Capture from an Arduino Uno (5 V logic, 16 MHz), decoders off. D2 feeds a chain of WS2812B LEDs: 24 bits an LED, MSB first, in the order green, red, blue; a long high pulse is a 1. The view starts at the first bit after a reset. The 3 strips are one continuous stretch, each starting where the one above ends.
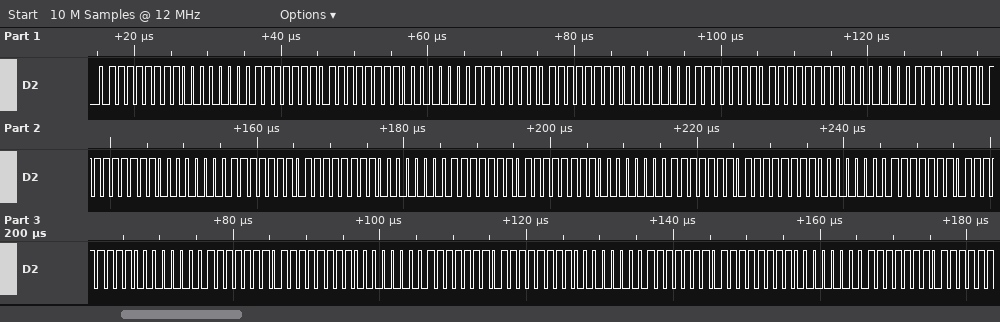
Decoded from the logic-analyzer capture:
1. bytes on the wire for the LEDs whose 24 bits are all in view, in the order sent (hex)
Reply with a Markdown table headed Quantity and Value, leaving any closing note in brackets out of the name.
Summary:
| Quantity | Value |
|---|---|
| bytes on the wire for the LEDs whose 24 bits are all in view, in the order sent | 7F 80 7F 7F 80 7F 7F 80 7F 7F 80 7F 7F 80 7F 7F 80 7F 7F 80 7F 7F 80 7F 7F 80 7F 7F 80 7F 7F 80 7F 7F 80 7F |
